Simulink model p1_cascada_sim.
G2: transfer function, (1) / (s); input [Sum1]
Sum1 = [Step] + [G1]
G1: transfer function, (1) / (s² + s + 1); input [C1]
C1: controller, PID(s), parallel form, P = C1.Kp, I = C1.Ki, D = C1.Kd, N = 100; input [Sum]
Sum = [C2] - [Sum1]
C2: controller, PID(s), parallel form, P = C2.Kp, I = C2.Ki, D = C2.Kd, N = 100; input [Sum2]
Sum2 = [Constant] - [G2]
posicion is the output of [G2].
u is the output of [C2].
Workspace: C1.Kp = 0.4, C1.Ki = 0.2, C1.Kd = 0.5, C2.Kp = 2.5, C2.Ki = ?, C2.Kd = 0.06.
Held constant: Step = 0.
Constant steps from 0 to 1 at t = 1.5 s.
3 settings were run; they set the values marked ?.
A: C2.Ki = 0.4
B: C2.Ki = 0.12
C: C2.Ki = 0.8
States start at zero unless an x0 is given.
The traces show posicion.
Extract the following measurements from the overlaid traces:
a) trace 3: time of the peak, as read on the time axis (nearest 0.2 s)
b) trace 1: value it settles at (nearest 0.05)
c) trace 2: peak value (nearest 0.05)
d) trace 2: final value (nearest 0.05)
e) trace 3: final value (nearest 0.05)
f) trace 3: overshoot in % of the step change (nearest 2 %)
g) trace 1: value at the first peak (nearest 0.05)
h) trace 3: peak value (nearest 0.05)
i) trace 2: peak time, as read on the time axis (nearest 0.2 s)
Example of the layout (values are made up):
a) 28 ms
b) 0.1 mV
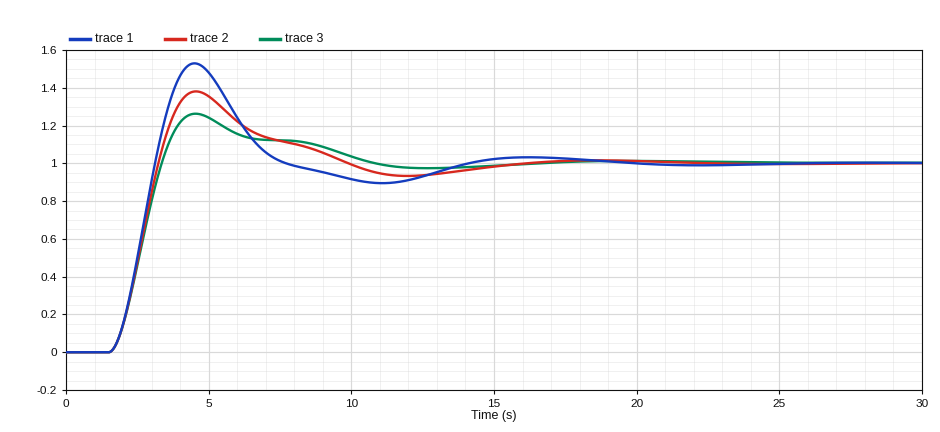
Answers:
a) 4.6 s
b) 1.00
c) 1.40
d) 1.00
e) 1.00
f) 26 %
g) 1.55
h) 1.25
i) 4.6 s
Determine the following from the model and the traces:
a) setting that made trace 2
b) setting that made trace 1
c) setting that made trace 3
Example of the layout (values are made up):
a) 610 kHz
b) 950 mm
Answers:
a) A
b) C
c) B
